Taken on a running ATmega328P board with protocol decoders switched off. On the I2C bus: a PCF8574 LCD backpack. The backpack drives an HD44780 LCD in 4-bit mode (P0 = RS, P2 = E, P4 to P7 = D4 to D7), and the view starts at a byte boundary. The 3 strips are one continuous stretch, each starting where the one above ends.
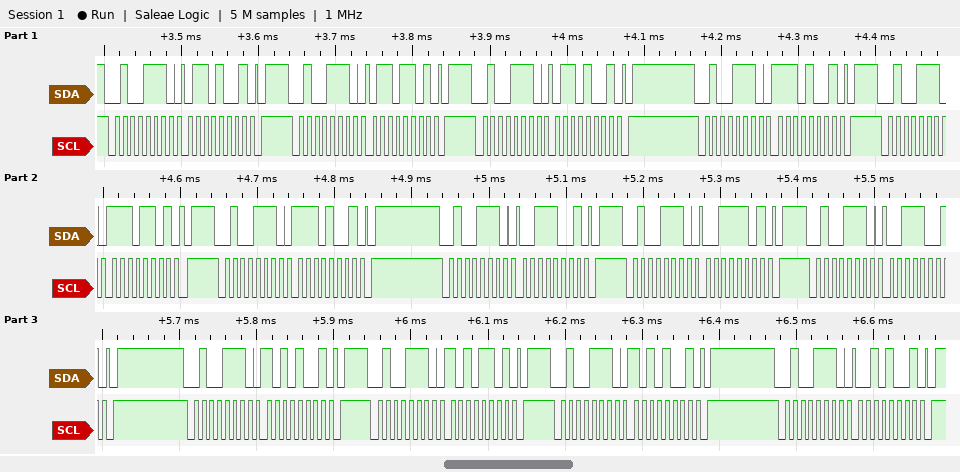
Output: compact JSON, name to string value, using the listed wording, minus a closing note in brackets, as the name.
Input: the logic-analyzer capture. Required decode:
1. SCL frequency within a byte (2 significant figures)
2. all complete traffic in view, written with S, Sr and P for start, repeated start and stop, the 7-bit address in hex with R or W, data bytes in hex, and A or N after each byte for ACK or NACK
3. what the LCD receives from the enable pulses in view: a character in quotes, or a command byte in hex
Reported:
{"SCL frequency within a byte": "100 kHz", "all complete traffic in view, written with S, Sr and P for start, repeated start and stop, the 7-bit address in hex with R or W, data bytes in hex, and A or N after each byte for ACK or NACK": "S 27W A 69 A P S 27W A 6D A P S 27W A 69 A P S 27W A E9 A P S 27W A ED A P S 27W A E9 A P S 27W A 39 A P S 27W A 3D A P S 27W A 39 A P S 27W A A9 A P S 27W A AD A P S 27W A A9 A P S 27W A 29 A P", "what the LCD receives from the enable pulses in view: a character in quotes, or a command byte in hex": "'n' ':'"}
